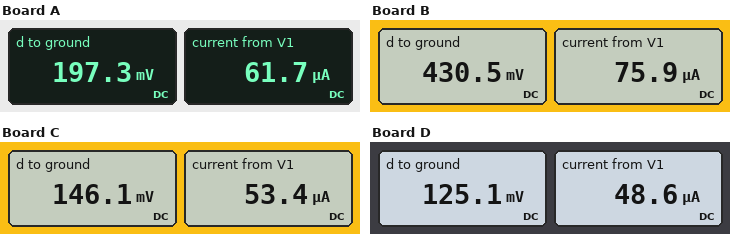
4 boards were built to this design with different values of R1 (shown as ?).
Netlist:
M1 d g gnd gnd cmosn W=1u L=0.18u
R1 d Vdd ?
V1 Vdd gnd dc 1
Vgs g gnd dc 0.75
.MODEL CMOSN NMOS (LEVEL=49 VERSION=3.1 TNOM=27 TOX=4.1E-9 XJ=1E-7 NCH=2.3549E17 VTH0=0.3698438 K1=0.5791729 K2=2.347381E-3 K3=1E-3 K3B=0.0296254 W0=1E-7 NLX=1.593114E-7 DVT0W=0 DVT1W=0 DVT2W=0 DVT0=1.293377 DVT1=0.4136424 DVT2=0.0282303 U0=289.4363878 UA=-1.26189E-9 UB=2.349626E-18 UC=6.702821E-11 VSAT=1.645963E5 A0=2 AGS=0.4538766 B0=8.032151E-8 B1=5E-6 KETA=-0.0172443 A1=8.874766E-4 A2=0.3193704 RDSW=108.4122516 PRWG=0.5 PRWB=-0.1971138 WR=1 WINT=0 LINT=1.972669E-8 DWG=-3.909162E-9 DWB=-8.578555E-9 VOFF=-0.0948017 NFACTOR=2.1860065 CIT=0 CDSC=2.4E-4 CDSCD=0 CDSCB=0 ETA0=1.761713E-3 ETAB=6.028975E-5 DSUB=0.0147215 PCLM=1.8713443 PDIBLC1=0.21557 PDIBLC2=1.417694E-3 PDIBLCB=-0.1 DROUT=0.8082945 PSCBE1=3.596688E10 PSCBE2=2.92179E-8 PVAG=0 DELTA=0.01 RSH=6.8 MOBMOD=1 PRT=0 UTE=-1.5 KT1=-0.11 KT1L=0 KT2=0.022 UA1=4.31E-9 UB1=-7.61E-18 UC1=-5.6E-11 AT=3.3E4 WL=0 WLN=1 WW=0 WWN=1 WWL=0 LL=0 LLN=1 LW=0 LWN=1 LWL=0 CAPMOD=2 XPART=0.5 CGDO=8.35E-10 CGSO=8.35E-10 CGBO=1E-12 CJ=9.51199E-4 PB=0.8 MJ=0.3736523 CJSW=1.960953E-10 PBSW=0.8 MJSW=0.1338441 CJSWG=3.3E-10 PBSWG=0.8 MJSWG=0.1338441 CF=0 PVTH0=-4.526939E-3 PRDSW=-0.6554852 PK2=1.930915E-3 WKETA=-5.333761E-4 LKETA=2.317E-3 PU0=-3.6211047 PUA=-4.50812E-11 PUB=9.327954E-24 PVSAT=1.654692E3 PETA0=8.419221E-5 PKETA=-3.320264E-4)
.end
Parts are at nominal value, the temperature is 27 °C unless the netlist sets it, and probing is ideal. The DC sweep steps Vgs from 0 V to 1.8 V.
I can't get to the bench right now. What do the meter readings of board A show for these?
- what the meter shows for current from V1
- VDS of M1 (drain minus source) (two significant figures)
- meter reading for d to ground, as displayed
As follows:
61.7 µA
200 mV
197.3 mV
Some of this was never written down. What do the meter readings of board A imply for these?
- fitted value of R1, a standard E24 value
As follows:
13 kΩ
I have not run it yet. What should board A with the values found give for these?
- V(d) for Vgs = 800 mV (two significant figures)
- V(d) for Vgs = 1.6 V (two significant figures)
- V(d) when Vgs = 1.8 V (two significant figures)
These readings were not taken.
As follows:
150 mV
48 mV
45 mV
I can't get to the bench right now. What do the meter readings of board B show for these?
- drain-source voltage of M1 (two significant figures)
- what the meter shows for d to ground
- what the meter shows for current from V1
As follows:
430 mV
430.5 mV
75.9 µA
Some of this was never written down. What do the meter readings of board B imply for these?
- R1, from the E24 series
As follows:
7.5 kΩ
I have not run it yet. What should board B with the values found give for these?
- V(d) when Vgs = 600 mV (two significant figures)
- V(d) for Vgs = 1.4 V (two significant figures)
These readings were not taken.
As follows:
790 mV
93 mV
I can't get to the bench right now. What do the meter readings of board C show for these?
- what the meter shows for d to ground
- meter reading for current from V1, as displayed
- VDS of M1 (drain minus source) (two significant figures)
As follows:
146.1 mV
53.4 µA
150 mV
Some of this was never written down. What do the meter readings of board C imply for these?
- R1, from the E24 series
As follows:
16 kΩ
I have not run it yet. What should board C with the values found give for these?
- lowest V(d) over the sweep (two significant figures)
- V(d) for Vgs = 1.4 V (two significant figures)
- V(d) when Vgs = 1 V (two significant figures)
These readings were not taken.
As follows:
37 mV
44 mV
68 mV
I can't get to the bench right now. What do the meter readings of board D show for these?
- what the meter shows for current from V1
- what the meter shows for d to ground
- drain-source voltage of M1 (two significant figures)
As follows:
48.6 µA
125.1 mV
130 mV
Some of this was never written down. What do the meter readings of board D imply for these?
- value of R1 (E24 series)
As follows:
18 kΩ
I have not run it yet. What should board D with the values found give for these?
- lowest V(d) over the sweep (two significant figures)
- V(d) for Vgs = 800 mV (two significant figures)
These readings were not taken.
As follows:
33 mV
99 mV
